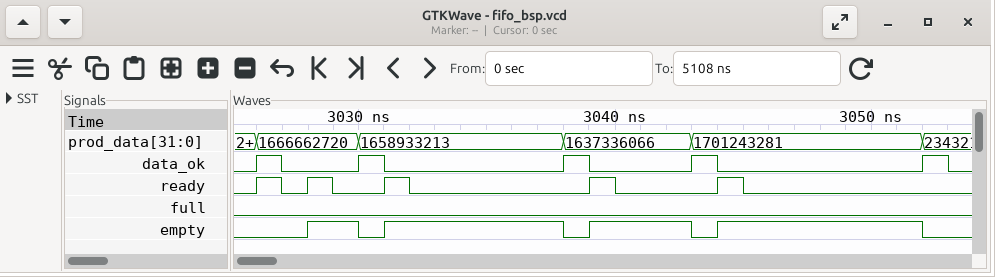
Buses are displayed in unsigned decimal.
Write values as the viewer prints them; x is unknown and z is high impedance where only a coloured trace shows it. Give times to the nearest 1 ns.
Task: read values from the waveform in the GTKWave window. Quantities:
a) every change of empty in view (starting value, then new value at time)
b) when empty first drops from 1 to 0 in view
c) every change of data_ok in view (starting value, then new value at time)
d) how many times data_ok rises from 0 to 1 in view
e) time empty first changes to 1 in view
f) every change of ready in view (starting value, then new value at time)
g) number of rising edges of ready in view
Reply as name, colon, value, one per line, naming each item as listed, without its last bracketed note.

every change of empty in view: 0, 1 at 3028 ns, 0 at 3030 ns, 1 at 3031 ns, 0 at 3038 ns, 1 at 3039 ns, 0 at 3043 ns, 1 at 3044 ns, 0 at 3052 ns
when empty first drops from 1 to 0 in view: 3030 ns
every change of data_ok in view: 0, 1 at 3026 ns, 0 at 3027 ns, 1 at 3030 ns, 0 at 3031 ns, 1 at 3038 ns, 0 at 3039 ns, 1 at 3043 ns, 0 at 3044 ns, 1 at 3052 ns, 0 at 3053 ns
how many times data_ok rises from 0 to 1 in view: 5
time empty first changes to 1 in view: 3028 ns
every change of ready in view: 0, 1 at 3026 ns, 0 at 3027 ns, 1 at 3028 ns, 0 at 3029 ns, 1 at 3031 ns, 0 at 3032 ns, 1 at 3039 ns, 0 at 3040 ns, 1 at 3044 ns, 0 at 3045 ns
number of rising edges of ready in view: 5
